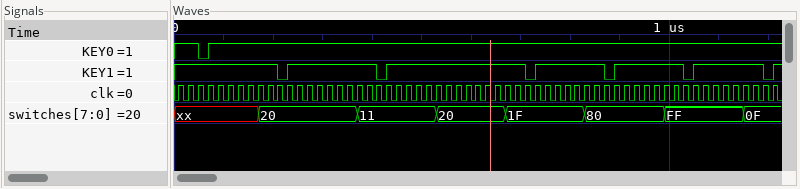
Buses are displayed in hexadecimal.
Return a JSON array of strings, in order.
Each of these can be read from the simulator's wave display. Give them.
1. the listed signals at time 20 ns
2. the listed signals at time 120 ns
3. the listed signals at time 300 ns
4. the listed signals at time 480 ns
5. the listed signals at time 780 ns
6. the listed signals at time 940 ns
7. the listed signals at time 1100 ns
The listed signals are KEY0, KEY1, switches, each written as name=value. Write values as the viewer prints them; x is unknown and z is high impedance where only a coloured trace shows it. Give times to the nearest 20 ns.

["KEY0=1, KEY1=1, switches=xx", "KEY0=1, KEY1=1, switches=xx", "KEY0=1, KEY1=1, switches=20", "KEY0=1, KEY1=1, switches=11", "KEY0=1, KEY1=1, switches=1F", "KEY0=1, KEY1=1, switches=80", "KEY0=1, KEY1=1, switches=FF"]
